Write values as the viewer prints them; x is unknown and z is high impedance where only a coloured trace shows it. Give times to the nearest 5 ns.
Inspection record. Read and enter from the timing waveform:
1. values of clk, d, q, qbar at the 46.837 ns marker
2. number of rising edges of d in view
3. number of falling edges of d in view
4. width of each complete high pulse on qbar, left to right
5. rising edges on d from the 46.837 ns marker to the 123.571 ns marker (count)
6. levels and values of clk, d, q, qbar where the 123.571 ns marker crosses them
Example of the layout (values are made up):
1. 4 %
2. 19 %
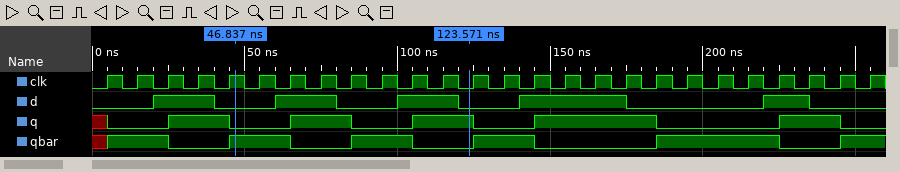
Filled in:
1. clk=1, d=0, q=0, qbar=1
2. 5
3. 5
4. 20 ns, 20 ns, 20 ns, 40 ns
5. 2
6. clk=0, d=0, q=1, qbar=0
